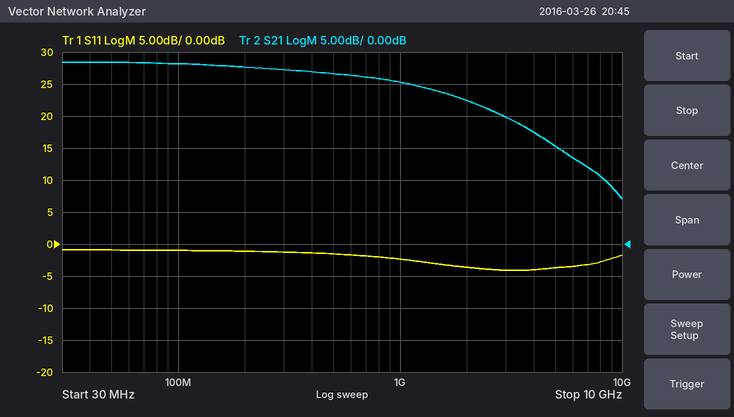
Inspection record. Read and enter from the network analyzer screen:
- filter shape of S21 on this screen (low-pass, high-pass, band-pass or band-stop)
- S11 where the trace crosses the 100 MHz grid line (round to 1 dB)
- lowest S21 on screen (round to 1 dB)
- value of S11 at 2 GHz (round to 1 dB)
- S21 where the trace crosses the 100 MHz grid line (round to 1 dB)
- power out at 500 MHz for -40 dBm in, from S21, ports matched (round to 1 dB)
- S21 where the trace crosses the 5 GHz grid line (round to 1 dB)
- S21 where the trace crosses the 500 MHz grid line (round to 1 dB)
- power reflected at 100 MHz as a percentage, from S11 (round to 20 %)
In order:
low-pass
-1 dB
7 dB
-4 dB
28 dB
-13 dBm
15 dB
27 dB
80 %
